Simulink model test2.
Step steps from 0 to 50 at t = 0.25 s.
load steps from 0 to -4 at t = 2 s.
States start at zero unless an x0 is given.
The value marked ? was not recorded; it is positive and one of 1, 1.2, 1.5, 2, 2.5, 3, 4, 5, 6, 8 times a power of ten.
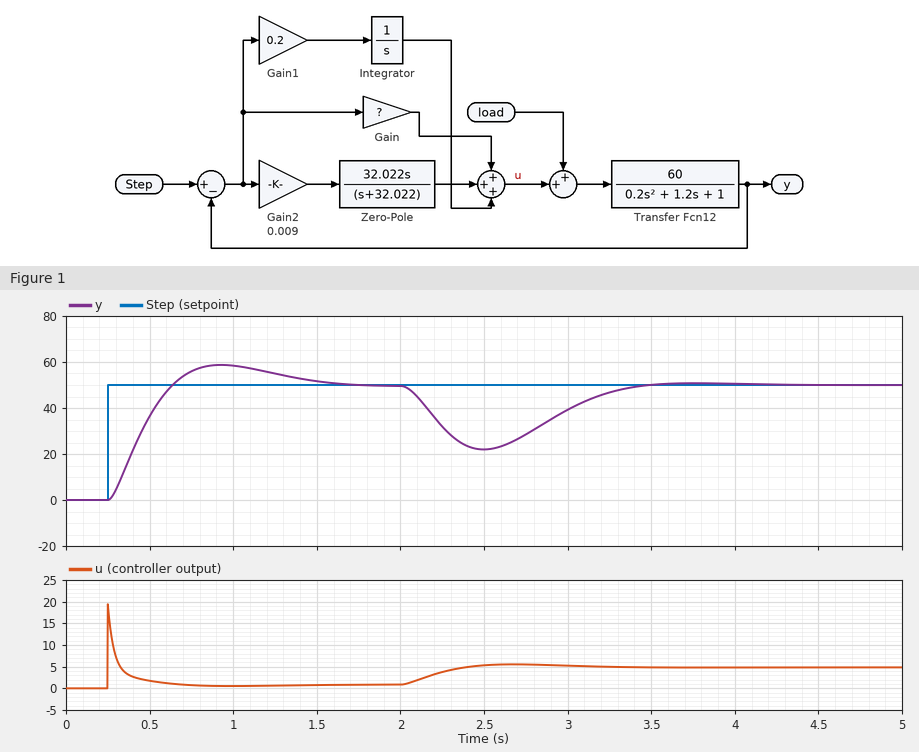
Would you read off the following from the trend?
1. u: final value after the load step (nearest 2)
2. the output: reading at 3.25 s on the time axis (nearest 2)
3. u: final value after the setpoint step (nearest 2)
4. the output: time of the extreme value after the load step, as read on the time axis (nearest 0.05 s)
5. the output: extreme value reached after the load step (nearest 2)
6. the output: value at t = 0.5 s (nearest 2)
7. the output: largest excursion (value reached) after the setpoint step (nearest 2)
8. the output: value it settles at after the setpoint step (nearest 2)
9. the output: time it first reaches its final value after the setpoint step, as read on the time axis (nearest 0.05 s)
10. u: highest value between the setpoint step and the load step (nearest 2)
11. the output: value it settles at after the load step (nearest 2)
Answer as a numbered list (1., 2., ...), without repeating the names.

1. 4
2. 46
3. 0
4. 2.50 s
5. 22
6. 36
7. 58
8. 50
9. 0.65 s
10. 20
11. 50
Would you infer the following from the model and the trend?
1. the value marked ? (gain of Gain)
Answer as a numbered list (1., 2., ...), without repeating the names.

1. 0.1
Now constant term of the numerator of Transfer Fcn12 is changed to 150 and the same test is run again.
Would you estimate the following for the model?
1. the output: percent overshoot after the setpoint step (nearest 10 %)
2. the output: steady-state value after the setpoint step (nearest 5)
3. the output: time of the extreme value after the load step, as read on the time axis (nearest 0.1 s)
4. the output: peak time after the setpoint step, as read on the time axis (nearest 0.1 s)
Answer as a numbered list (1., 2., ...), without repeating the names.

1. 20 %
2. 50
3. 2.3 s
4. 0.6 s
